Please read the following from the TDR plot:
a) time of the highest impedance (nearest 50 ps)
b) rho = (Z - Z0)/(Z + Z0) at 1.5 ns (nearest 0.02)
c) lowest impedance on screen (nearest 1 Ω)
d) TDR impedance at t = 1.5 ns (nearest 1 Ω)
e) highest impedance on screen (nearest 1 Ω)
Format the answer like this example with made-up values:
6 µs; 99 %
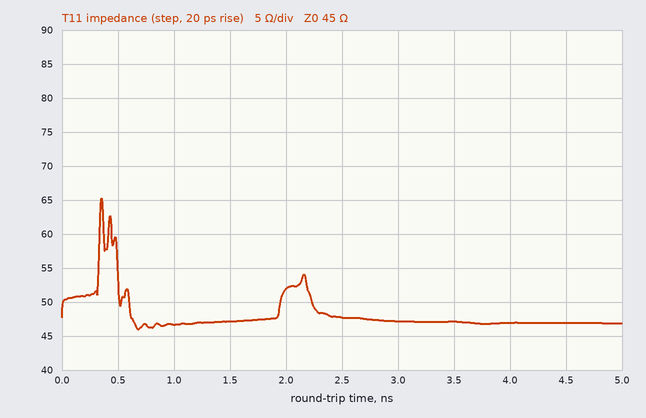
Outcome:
350 ps; +0.02; 46 Ω; 47 Ω; 65 Ω
